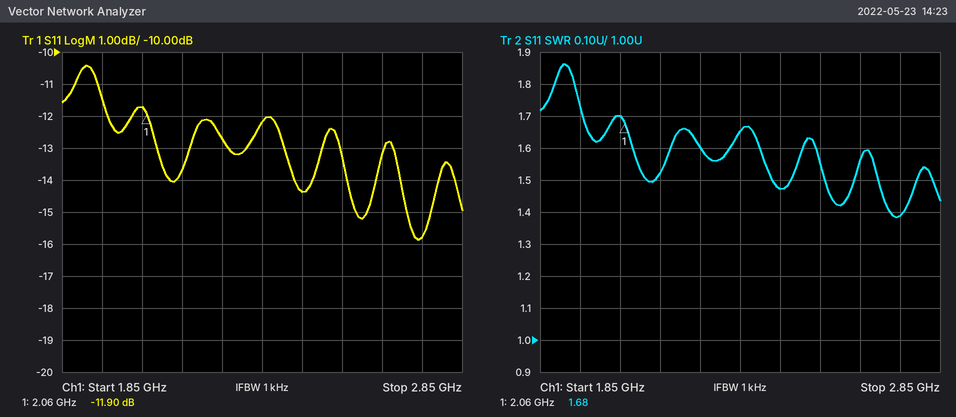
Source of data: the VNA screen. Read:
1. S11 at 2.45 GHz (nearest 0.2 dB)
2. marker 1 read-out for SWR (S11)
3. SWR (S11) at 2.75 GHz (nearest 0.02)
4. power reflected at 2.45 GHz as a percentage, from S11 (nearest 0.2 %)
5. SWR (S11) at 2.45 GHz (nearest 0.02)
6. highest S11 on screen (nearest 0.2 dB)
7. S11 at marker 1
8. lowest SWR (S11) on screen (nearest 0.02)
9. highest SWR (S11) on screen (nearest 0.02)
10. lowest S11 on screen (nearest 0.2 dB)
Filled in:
-14.4 dB
1.68
1.38
3.6 %
1.48
-10.4 dB
-11.90 dB
1.38
1.86
-15.8 dB
